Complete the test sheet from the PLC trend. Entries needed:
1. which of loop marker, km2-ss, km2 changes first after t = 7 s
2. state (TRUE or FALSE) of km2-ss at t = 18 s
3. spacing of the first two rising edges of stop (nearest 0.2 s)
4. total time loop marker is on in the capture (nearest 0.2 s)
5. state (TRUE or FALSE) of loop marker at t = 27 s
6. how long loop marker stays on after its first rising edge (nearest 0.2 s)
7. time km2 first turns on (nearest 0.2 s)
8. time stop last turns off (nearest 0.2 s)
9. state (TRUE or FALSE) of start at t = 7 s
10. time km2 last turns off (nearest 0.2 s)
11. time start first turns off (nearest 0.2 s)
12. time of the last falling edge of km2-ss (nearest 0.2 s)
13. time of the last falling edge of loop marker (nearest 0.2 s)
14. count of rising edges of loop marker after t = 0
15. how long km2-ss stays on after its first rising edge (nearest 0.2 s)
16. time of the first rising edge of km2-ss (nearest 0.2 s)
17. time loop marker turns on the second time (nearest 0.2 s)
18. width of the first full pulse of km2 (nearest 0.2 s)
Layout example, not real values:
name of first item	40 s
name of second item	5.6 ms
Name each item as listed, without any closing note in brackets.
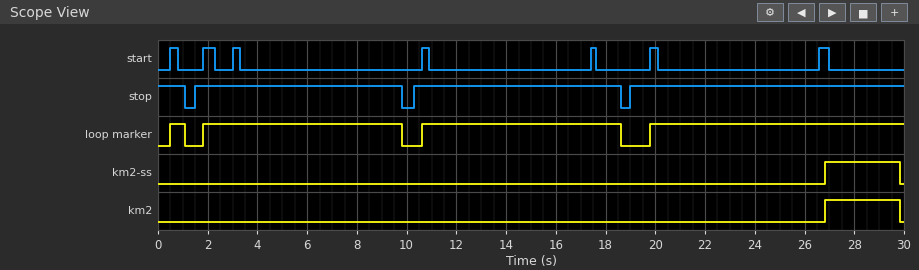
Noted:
which of loop marker, km2-ss, km2 changes first after t = 7 s	loop marker
state (TRUE or FALSE) of km2-ss at t = 18 s	FALSE
spacing of the first two rising edges of stop	8.8 s
total time loop marker is on in the capture	26.8 s
state (TRUE or FALSE) of loop marker at t = 27 s	TRUE
how long loop marker stays on after its first rising edge	0.6 s
time km2 first turns on	26.8 s
time stop last turns off	18.6 s
state (TRUE or FALSE) of start at t = 7 s	FALSE
time km2 last turns off	29.8 s
time start first turns off	0.8 s
time of the last falling edge of km2-ss	29.8 s
time of the last falling edge of loop marker	18.6 s
count of rising edges of loop marker after t = 0	4
how long km2-ss stays on after its first rising edge	3.0 s
time of the first rising edge of km2-ss	26.8 s
time loop marker turns on the second time	1.8 s
width of the first full pulse of km2	3.0 s
